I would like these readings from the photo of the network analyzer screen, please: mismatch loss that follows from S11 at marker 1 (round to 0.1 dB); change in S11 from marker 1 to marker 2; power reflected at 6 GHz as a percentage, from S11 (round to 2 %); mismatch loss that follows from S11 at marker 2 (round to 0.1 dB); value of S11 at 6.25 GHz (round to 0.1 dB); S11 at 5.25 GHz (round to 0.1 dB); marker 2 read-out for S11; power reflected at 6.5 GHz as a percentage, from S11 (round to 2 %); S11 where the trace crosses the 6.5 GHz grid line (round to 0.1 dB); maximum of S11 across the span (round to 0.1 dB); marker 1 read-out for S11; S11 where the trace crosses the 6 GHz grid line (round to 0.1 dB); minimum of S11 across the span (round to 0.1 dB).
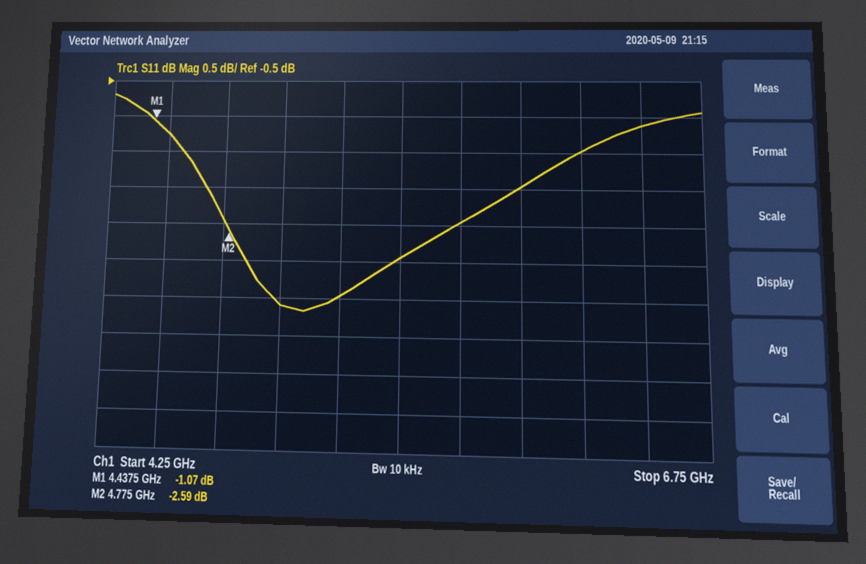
6.6 dB
-1.52 dB
64 %
3.5 dB
-1.5 dB
-3.5 dB
-2.59 dB
78 %
-1.1 dB
-0.7 dB
-1.07 dB
-2.0 dB
-3.7 dB
